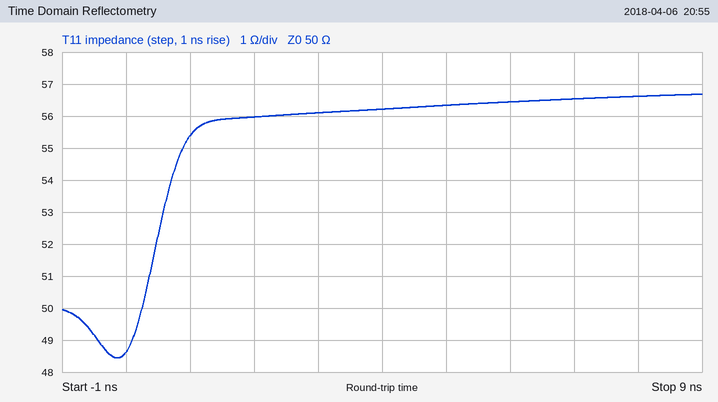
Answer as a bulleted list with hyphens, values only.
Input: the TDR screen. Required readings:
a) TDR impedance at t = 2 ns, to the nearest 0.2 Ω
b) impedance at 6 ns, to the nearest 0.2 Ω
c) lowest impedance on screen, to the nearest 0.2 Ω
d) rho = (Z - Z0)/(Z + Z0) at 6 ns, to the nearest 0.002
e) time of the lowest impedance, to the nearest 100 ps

- 56.0 Ω
- 56.4 Ω
- 48.4 Ω
- +0.060
- -100 ps
